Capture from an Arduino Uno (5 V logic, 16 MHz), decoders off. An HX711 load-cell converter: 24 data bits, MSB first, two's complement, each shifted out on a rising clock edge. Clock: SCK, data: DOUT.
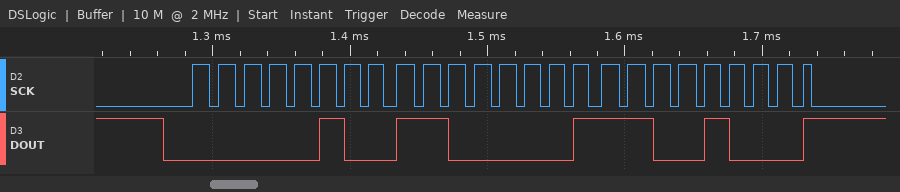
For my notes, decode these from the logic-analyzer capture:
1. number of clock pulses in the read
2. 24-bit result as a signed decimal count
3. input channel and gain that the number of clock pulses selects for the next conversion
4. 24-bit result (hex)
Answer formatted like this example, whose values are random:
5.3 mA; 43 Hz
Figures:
25; 311752; channel A, gain 128; 0x04C1C8
